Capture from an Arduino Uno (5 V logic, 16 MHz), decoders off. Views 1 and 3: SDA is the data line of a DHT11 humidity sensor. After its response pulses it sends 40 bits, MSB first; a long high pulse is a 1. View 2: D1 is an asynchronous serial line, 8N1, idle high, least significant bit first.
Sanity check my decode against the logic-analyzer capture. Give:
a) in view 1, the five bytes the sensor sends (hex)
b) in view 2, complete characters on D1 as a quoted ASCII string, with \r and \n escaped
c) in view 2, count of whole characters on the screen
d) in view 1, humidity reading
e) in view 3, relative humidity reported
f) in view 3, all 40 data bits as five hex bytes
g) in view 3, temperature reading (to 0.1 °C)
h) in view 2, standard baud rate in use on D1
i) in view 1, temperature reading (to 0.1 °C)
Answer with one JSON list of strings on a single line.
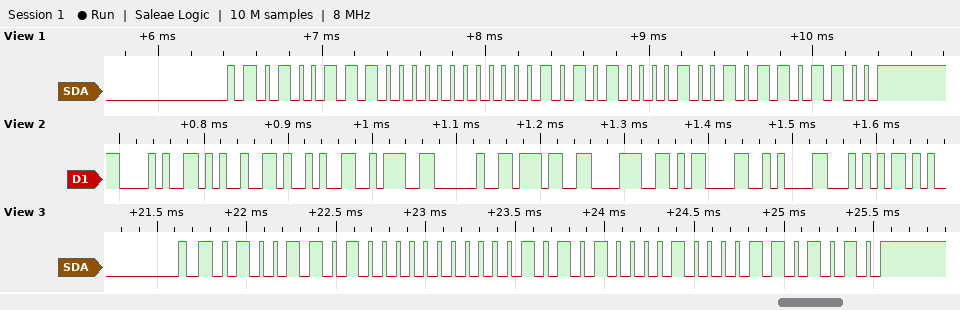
["4E 00 15 09 6C", "\"(%): 78\\r\\nT\"", "10", "78 %", "77 %", "4D 00 15 08 6A", "21.8 °C", "115200 baud", "21.9 °C"]
